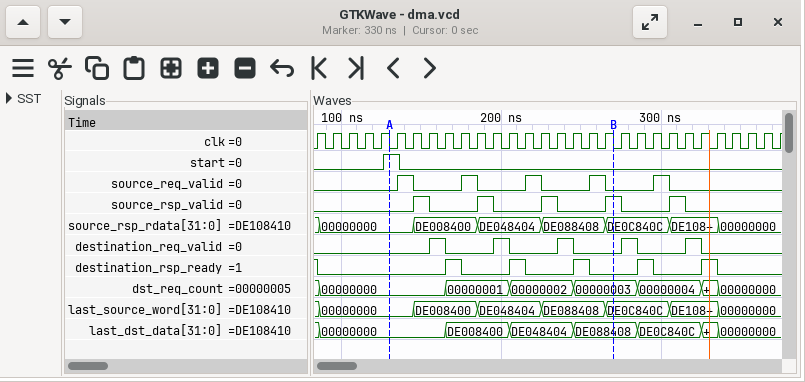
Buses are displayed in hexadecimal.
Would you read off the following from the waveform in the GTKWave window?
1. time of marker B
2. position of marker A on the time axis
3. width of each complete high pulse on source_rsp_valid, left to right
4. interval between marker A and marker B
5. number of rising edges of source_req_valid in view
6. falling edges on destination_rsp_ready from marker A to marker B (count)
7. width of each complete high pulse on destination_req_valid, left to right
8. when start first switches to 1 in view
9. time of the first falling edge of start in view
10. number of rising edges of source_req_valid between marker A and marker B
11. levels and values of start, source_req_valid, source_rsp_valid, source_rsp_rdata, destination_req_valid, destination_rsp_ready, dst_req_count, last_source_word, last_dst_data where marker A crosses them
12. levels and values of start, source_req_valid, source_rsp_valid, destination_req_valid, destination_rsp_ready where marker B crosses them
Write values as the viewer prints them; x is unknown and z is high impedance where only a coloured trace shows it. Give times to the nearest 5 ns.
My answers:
270 ns
130 ns
10 ns, 10 ns, 10 ns, 10 ns, 10 ns
140 ns
5
3
10 ns, 10 ns, 10 ns, 10 ns, 10 ns
125 ns
135 ns
4
start=1, source_req_valid=0, source_rsp_valid=0, source_rsp_rdata=00000000, destination_req_valid=0, destination_rsp_ready=0, dst_req_count=00000000, last_source_word=00000000, last_dst_data=00000000
start=0, source_req_valid=0, source_rsp_valid=1, destination_req_valid=0, destination_rsp_ready=0
